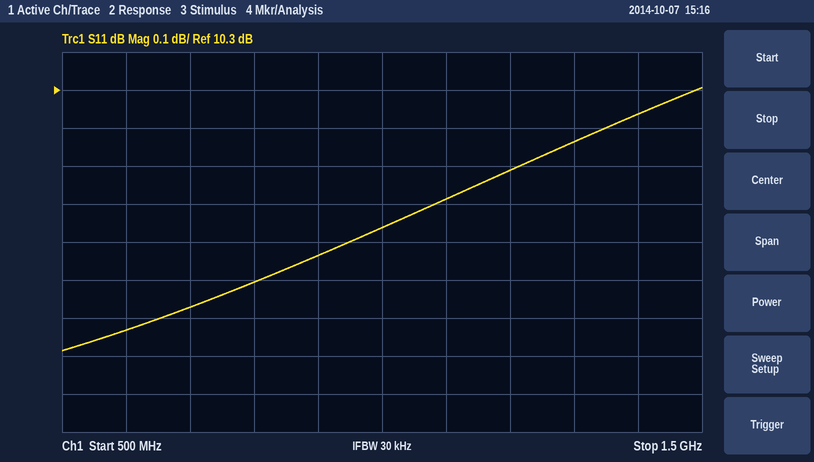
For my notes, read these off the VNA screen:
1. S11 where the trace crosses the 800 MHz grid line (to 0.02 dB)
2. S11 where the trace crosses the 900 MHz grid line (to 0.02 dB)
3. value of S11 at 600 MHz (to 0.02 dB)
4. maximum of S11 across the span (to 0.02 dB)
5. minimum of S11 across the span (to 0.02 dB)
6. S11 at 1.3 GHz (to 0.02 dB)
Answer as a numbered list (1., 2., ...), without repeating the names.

1. 9.80 dB
2. 9.86 dB
3. 9.66 dB
4. 10.30 dB
5. 9.62 dB
6. 10.16 dB
